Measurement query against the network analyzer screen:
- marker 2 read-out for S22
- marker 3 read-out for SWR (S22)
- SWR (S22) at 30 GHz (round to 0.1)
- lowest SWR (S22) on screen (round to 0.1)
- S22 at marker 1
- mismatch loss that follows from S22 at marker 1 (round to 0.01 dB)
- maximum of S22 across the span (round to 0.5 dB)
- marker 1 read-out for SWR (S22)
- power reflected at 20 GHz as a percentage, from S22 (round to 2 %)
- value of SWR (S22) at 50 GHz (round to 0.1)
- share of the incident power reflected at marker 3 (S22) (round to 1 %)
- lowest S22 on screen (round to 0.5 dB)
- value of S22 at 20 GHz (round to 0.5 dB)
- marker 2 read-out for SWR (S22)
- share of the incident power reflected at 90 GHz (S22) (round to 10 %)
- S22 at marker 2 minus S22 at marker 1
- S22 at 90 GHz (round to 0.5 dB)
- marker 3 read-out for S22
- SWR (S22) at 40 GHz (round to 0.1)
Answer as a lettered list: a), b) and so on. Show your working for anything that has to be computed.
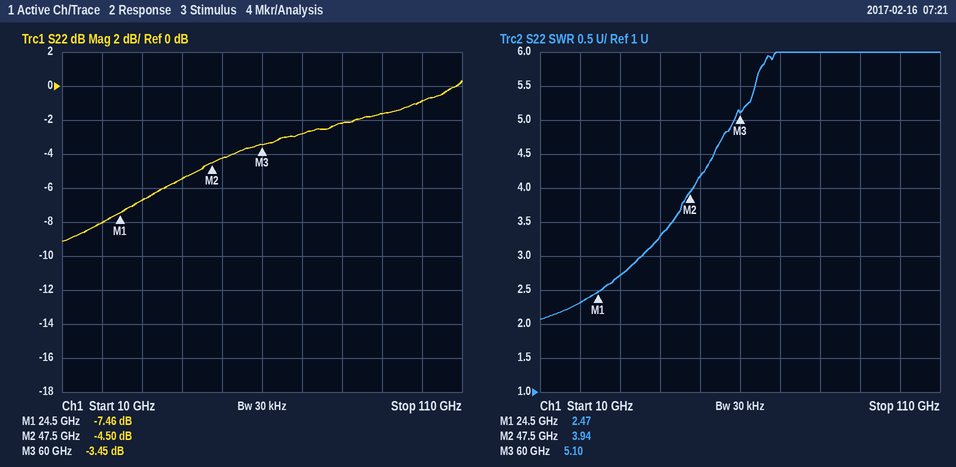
a) -4.50 dB
b) 5.10
c) 2.7
d) 2.1
e) -7.46 dB
f) −10 log10(1 − 10^(-7.46/10)) ≈ 0.86 dB
g) 0.5 dB
h) 2.47
i) 10^(-8/10) ≈ 16 %
j) 4.2
k) 10^(-3.45/10) ≈ 45 %
l) -9.0 dB
m) -8.0 dB
n) 3.94
o) 10^(-1.5/10) ≈ 70.8 %, so 70 % to the nearest 10 %
p) -4.5 − (-7.46) = 2.96 dB
q) -1.5 dB
r) -3.45 dB
s) 3.3
